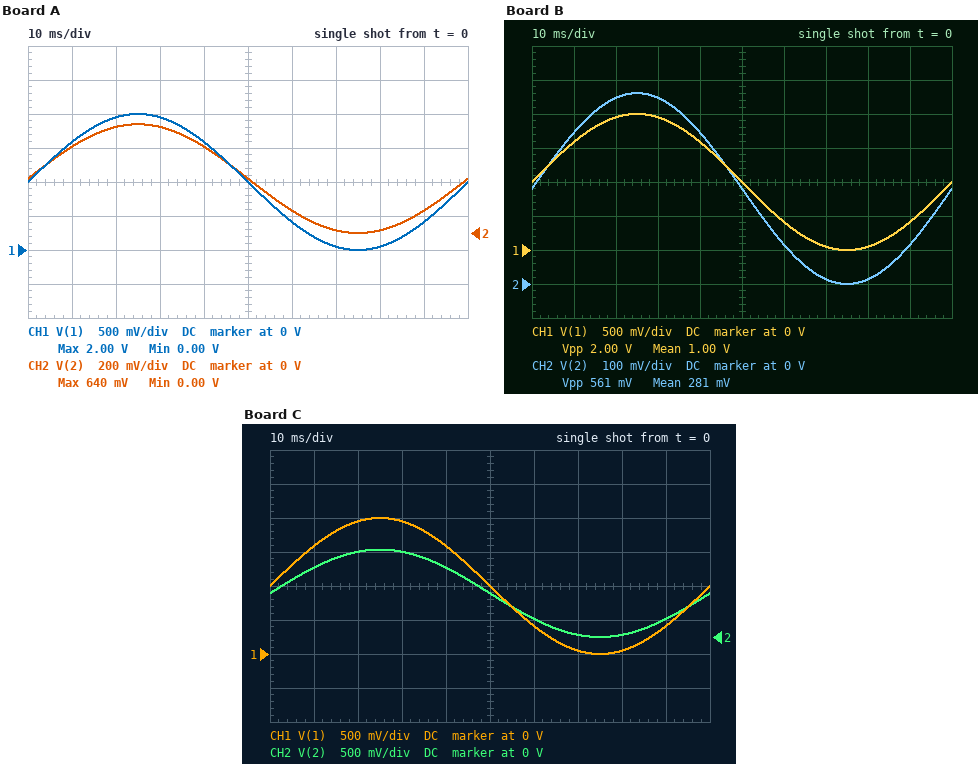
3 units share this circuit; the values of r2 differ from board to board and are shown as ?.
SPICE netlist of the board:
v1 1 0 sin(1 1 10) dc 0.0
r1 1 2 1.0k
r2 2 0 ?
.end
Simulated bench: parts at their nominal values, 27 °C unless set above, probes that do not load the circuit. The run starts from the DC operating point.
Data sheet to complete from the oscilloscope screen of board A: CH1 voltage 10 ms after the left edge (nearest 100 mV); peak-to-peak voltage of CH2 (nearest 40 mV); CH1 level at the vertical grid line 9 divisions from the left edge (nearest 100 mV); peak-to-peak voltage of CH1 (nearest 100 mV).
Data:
1.6 V
640 mV
400 mV
2.0 V
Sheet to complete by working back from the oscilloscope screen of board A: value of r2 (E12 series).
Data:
470 Ω
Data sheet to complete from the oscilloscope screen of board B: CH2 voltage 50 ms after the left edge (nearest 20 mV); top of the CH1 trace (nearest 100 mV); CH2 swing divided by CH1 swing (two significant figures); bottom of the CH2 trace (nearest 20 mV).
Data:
280 mV
2.0 V
0.28
0 V
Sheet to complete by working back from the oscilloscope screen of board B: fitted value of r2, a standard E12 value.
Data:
390 Ω
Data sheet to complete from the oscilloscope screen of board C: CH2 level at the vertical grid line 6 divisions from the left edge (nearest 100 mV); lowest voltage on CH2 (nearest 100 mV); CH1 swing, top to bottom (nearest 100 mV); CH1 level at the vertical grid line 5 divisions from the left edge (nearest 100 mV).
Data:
300 mV
0 V
2.0 V
1.0 V
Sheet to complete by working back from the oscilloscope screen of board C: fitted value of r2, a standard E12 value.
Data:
1.8 kΩ
